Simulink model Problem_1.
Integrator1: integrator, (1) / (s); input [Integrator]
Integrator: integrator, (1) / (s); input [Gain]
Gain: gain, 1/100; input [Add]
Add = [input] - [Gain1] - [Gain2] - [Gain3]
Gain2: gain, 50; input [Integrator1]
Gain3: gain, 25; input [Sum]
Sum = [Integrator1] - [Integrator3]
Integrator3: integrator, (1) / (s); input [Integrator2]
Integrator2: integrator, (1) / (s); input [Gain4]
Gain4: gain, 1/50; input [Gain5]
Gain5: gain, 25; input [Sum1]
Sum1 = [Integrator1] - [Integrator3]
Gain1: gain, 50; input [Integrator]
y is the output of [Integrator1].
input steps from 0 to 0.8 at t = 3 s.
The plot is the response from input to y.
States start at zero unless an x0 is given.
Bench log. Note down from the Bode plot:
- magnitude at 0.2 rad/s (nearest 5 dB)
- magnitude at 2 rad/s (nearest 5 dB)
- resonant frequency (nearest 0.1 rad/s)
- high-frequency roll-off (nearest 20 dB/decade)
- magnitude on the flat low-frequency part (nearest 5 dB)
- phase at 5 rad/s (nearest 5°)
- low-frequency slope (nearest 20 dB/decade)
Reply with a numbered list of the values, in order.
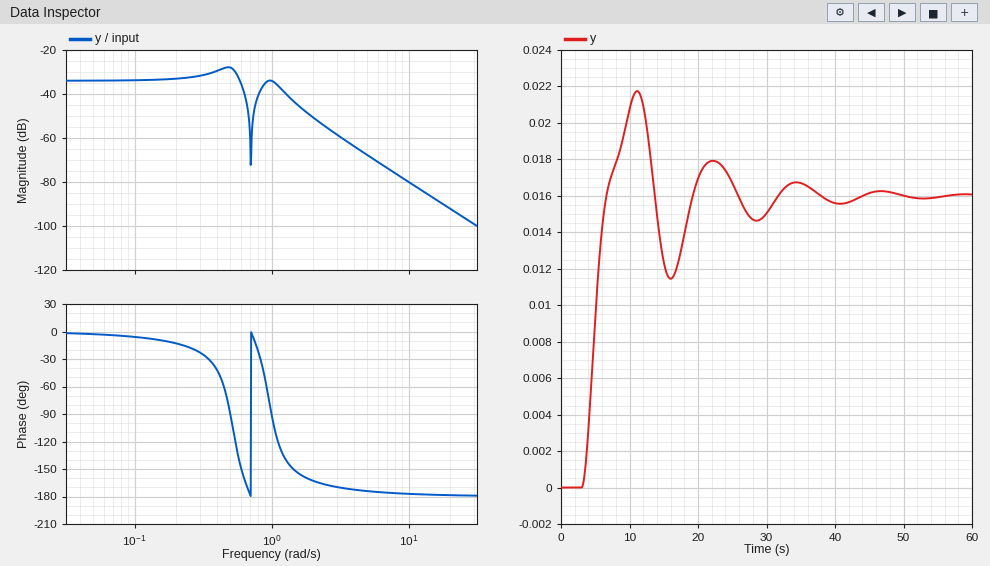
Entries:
1. -35 dB
2. -50 dB
3. 0.5 rad/s
4. -40 dB/decade
5. -35 dB
6. -175°
7. 0 dB/decade
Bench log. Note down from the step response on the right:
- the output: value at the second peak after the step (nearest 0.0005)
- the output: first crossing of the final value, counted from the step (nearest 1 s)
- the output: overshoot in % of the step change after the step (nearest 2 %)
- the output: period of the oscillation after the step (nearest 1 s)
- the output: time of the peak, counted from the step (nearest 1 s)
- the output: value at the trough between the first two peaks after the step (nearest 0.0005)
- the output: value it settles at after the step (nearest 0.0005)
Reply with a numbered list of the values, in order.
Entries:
1. 0.0180
2. 4 s
3. 36 %
4. 11 s
5. 8 s
6. 0.0115
7. 0.0160
